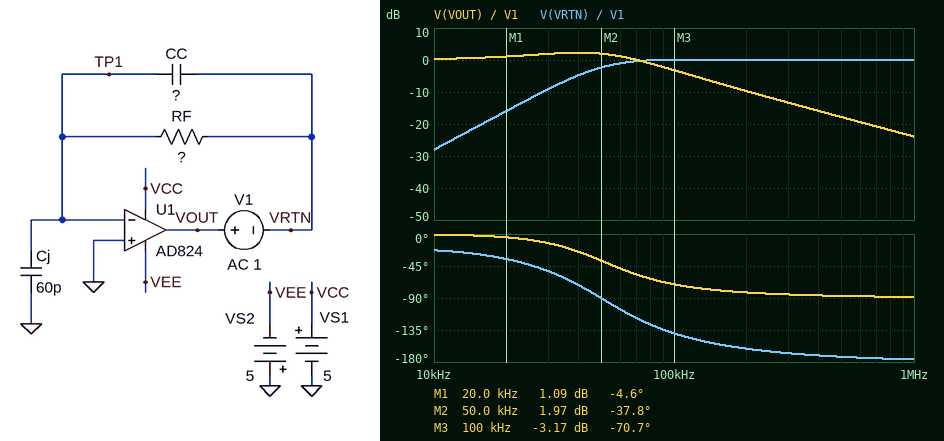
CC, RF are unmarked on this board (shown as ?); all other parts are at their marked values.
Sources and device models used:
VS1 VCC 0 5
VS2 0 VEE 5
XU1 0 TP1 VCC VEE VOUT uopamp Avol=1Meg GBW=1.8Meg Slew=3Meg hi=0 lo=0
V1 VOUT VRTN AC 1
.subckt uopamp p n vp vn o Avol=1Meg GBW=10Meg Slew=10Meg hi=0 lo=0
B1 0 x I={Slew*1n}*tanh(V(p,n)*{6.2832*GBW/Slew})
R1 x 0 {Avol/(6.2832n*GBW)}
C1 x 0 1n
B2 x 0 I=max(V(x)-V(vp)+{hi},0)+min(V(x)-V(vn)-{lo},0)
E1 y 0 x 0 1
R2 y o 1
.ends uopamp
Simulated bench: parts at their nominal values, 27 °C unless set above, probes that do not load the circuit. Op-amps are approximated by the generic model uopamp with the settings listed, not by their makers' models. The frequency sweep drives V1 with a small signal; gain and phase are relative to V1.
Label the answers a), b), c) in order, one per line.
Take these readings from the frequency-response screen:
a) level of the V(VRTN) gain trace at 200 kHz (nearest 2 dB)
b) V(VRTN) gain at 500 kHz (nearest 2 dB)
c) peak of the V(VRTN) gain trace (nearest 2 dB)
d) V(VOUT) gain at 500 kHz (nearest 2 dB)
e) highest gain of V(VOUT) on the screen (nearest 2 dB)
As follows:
a) 0 dB
b) 0 dB
c) 0 dB
d) -18 dB
e) 2 dB
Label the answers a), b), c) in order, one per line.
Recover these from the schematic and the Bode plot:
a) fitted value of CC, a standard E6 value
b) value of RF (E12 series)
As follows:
a) 2.2 pF
b) 1.8 MΩ
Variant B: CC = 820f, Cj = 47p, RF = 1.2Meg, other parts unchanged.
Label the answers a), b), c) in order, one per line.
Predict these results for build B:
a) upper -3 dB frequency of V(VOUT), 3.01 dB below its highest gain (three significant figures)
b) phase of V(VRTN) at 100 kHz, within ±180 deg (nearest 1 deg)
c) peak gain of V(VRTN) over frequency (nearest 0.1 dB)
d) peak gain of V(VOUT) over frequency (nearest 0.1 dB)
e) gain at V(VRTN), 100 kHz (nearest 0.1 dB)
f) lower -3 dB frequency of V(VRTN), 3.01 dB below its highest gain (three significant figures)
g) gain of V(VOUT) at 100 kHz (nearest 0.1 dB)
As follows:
a) 83.1 kHz
b) -148 deg
c) 6.7 dB
d) 7.4 dB
e) 4.4 dB
f) 60.8 kHz
g) -0.2 dB
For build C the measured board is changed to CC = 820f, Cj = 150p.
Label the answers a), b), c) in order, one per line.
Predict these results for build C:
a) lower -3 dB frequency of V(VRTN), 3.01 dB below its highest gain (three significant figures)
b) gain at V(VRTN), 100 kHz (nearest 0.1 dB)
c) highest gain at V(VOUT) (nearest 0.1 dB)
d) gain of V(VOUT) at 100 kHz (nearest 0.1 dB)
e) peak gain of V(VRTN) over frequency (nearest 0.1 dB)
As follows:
a) 28.9 kHz
b) 0.9 dB
c) 10.4 dB
d) -15.9 dB
e) 10.0 dB
